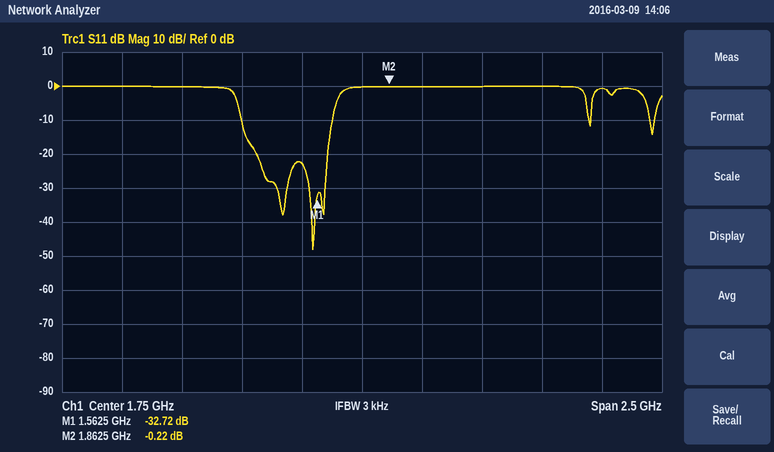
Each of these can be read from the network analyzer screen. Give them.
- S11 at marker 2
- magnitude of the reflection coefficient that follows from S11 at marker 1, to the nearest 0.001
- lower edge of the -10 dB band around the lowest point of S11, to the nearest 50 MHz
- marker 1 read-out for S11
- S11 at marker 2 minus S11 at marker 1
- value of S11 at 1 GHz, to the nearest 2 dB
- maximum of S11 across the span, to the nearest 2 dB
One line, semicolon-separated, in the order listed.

-0.22 dB; 0.023; 1.25 GHz; -32.72 dB; 32.50 dB; 0 dB; 0 dB
